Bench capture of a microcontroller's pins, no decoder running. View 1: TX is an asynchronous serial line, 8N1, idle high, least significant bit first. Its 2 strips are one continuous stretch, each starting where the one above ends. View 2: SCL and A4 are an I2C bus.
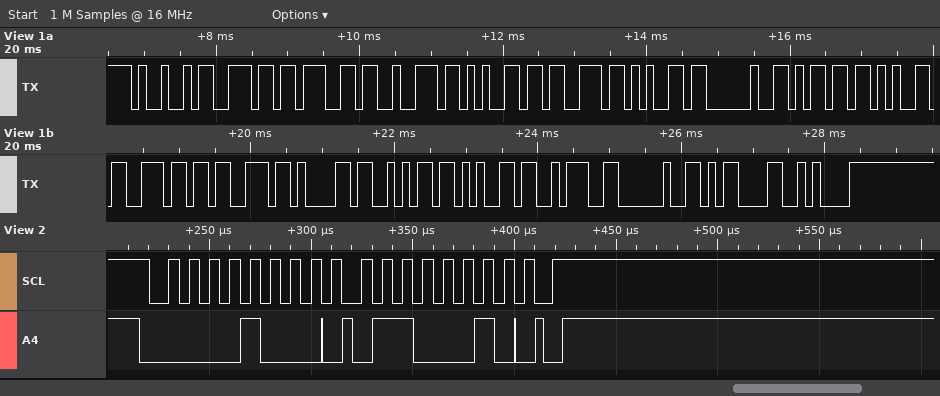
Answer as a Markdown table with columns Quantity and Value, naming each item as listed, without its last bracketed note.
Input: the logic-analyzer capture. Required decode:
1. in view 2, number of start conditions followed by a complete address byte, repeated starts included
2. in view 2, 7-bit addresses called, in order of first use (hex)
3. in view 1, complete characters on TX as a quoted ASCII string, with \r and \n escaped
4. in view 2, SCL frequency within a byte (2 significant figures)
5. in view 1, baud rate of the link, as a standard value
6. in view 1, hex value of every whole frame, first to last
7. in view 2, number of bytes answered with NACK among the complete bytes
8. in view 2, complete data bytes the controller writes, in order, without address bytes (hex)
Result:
| Quantity | Value |
|---|---|
| in view 2, number of start conditions followed by a complete address byte, repeated starts included | 1 |
| in view 2, 7-bit addresses called, in order of first use | 0x04 |
| in view 1, complete characters on TX as a quoted ASCII string, with \r and \n escaped | "Ingrese mensaje: \r\n" |
| in view 2, SCL frequency within a byte | 100 kHz |
| in view 1, baud rate of the link, as a standard value | 9600 baud |
| in view 1, hex value of every whole frame, first to last | 0x49 0x6E 0x67 0x72 0x65 0x73 0x65 0x20 0x6D 0x65 0x6E 0x73 0x61 0x6A 0x65 0x3A 0x20 0x0D 0x0A |
| in view 2, number of bytes answered with NACK among the complete bytes | 0 |
| in view 2, complete data bytes the controller writes, in order, without address bytes | 62 |
